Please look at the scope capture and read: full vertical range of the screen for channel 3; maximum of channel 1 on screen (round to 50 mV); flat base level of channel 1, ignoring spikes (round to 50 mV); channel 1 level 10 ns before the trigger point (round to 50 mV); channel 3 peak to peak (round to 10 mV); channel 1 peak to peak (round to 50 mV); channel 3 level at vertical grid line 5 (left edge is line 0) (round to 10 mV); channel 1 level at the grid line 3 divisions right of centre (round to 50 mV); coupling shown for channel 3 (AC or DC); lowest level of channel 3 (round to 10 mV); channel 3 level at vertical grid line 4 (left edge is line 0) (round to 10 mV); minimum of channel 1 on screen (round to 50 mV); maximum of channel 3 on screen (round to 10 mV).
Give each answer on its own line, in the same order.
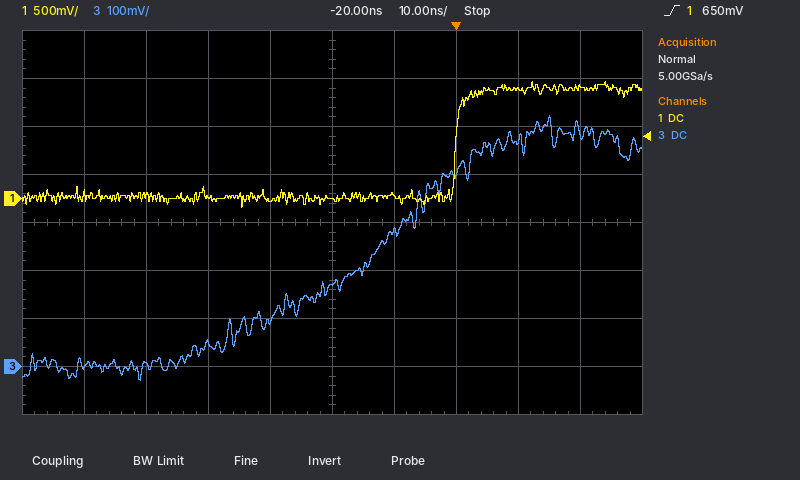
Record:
800 mV
1.20 V
0 mV
50 mV
550 mV
1.30 V
170 mV
1.15 V
DC
-30 mV
100 mV
-100 mV
520 mV
